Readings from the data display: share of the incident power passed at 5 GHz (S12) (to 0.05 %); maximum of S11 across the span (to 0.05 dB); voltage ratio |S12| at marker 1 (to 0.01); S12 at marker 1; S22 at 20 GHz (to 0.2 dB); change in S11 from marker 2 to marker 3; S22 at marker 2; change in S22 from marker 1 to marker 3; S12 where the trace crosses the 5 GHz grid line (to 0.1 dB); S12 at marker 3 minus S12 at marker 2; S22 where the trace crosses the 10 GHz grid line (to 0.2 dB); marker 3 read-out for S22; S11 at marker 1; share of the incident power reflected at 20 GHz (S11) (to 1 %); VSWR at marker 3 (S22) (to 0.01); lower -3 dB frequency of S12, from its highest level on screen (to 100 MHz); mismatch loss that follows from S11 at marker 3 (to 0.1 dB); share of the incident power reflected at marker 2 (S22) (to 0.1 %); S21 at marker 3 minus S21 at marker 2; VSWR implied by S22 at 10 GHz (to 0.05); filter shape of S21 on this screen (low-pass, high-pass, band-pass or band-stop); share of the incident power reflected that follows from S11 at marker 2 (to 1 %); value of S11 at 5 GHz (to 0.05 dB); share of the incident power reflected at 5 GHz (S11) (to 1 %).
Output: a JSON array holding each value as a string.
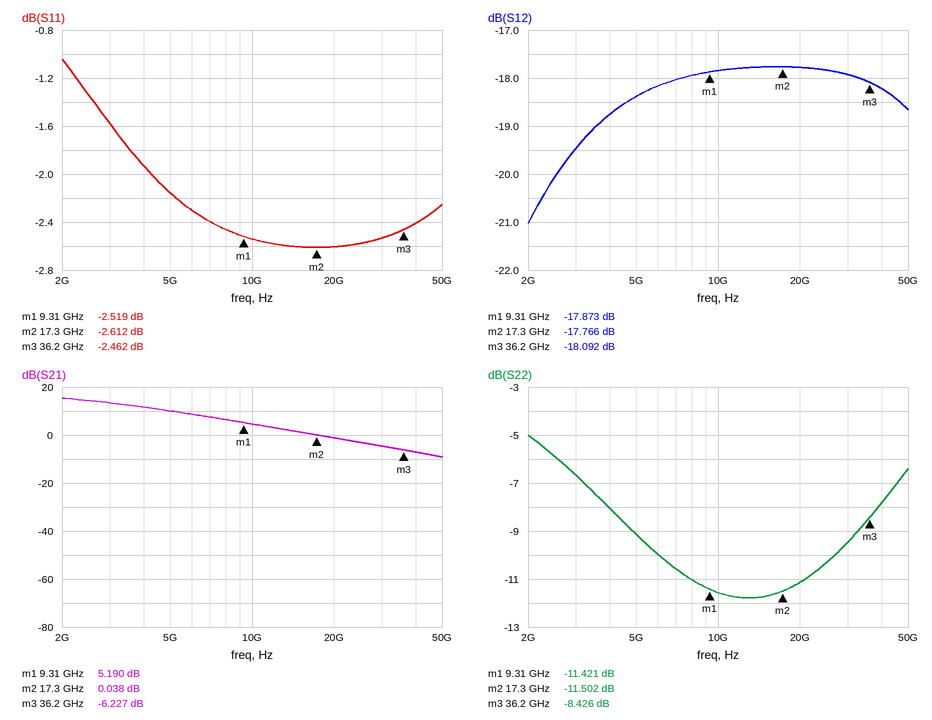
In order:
["1.45 %", "-1.05 dB", "0.13", "-17.873 dB", "-11.2 dB", "0.150 dB", "-11.502 dB", "2.995 dB", "-18.4 dB", "-0.326 dB", "-11.6 dB", "-8.426 dB", "-2.519 dB", "55 %", "2.22", "2.1 GHz", "3.6 dB", "7.1 %", "-6.265 dB", "1.70", "low-pass", "55 %", "-2.15 dB", "61 %"]
